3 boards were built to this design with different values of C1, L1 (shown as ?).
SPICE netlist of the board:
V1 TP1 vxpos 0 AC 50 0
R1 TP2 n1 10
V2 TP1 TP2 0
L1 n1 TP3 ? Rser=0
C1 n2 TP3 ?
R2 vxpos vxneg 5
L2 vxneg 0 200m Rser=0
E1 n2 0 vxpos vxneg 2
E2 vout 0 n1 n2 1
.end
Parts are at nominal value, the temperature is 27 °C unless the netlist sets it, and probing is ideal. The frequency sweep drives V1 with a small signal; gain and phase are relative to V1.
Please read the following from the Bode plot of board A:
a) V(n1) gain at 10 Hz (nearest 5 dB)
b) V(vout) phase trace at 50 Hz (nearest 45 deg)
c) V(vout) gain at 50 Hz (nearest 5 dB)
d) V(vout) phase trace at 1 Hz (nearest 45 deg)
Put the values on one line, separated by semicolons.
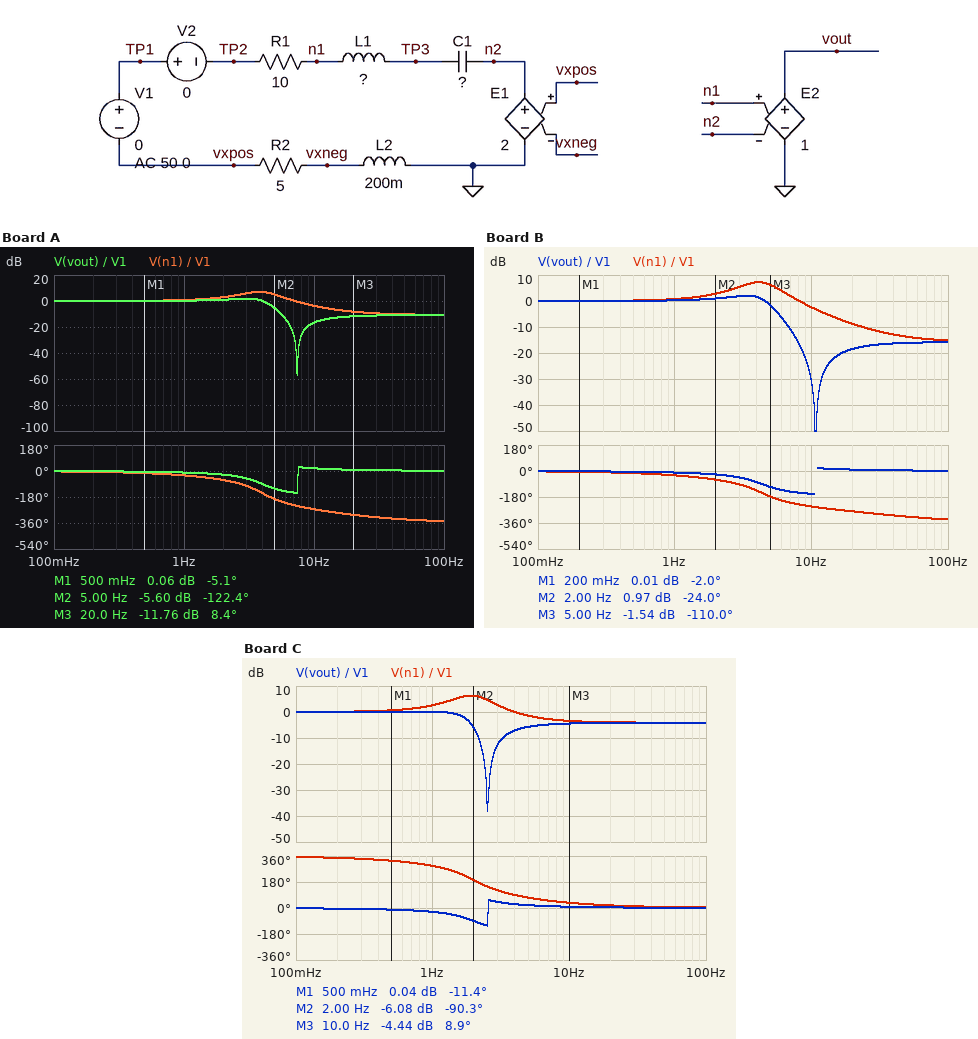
-5 dB; 0 deg; -10 dB; 0 deg
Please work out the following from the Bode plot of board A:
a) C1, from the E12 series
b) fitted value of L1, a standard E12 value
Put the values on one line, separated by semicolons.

5.6 mF; 82 mH
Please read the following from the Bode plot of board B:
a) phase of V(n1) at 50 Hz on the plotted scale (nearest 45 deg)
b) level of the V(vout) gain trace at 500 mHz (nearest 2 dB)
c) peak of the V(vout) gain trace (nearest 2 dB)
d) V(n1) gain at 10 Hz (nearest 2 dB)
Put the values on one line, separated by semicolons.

-315 deg; 0 dB; 2 dB; -2 dB
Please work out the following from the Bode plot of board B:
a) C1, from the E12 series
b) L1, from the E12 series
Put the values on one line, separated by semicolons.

5.6 mF; 39 mH
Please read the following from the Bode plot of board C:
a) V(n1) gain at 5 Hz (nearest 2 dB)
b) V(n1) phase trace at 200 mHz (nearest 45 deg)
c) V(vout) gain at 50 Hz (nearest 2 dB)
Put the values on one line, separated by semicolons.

-2 dB; 360 deg; -4 dB
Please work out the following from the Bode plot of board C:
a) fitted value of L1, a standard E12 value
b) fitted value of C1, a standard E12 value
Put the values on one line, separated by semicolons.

330 mH; 12 mF
